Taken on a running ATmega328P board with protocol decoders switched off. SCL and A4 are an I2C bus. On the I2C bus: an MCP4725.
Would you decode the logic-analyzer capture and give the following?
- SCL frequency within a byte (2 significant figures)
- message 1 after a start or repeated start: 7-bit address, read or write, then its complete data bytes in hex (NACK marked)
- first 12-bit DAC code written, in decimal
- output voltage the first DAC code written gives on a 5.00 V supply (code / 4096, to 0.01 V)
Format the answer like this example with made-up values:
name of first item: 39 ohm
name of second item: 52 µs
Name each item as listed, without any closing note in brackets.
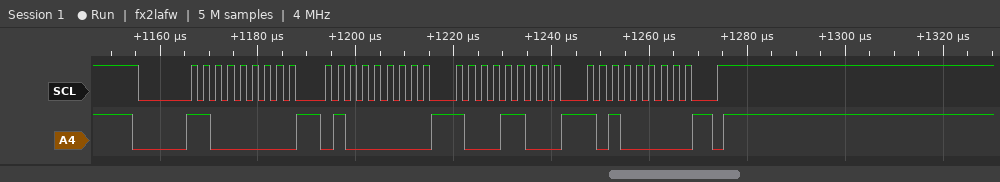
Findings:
SCL frequency within a byte: 400 kHz
message 1 after a start or repeated start: 7-bit address, read or write, then its complete data bytes in hex: 0x60 write: 40 8C A0
first 12-bit DAC code written, in decimal: 2250
output voltage the first DAC code written gives on a 5.00 V supply: 2.75 V
